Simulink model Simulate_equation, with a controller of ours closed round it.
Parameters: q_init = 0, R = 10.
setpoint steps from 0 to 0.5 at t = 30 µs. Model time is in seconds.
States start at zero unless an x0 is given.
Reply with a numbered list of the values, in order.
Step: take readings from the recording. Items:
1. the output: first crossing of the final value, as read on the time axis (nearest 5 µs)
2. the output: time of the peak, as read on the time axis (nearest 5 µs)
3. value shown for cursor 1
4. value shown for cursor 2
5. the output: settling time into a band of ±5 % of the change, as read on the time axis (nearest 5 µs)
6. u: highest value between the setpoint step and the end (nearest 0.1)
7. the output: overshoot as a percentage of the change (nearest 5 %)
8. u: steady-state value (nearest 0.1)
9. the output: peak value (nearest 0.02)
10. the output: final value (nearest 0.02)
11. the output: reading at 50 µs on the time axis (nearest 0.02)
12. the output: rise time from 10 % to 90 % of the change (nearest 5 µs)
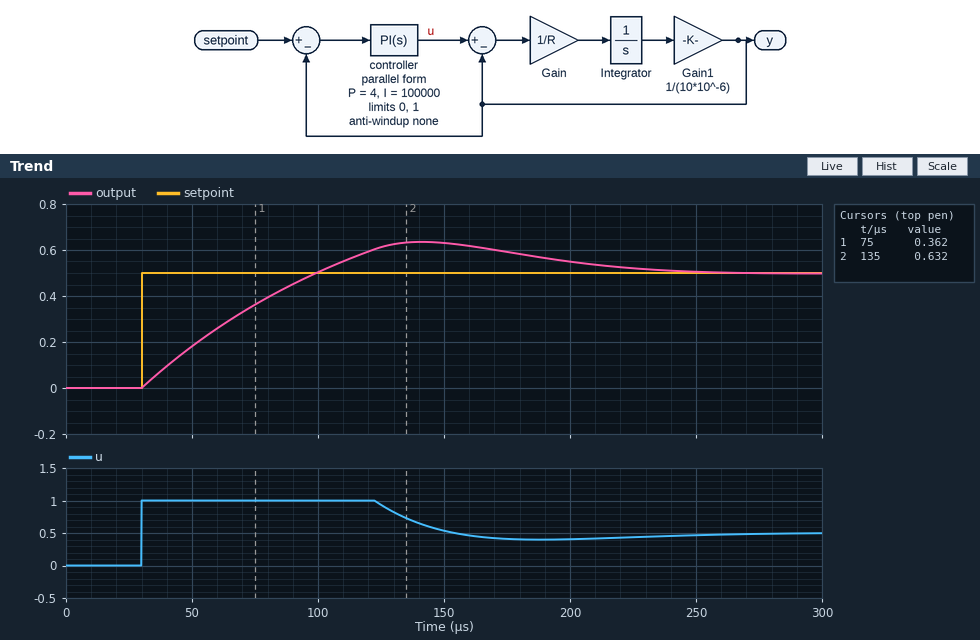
1. 100 µs
2. 140 µs
3. 0.362
4. 0.632
5. 220 µs
6. 1.0
7. 25 %
8. 0.5
9. 0.64
10. 0.50
11. 0.18
12. 55 µs
